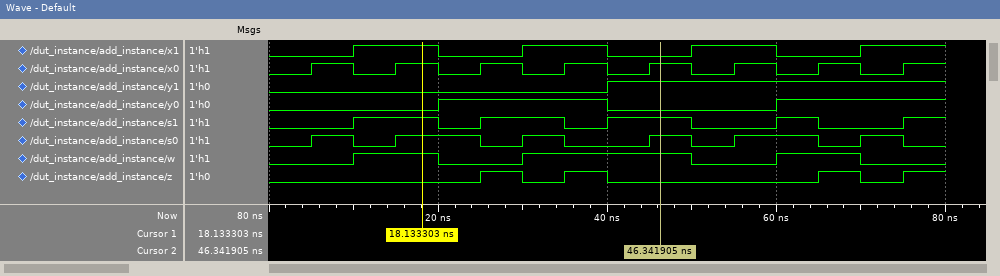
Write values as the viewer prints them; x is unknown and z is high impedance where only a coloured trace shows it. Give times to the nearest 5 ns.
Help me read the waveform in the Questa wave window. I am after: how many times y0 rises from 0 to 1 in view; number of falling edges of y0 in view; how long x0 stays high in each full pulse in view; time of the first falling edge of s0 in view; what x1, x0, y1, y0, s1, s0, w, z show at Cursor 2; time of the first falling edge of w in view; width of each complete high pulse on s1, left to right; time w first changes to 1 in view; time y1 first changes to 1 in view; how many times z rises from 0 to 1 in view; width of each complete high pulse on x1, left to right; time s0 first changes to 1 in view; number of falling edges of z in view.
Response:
2
1
5 ns, 5 ns, 5 ns, 5 ns, 5 ns, 5 ns, 5 ns
10 ns
x1=0, x0=1, y1=1, y0=0, s1=1, s0=1, w=1, z=0
20 ns
10 ns, 10 ns, 10 ns, 5 ns
10 ns
40 ns
4
10 ns, 10 ns, 10 ns
5 ns
3
